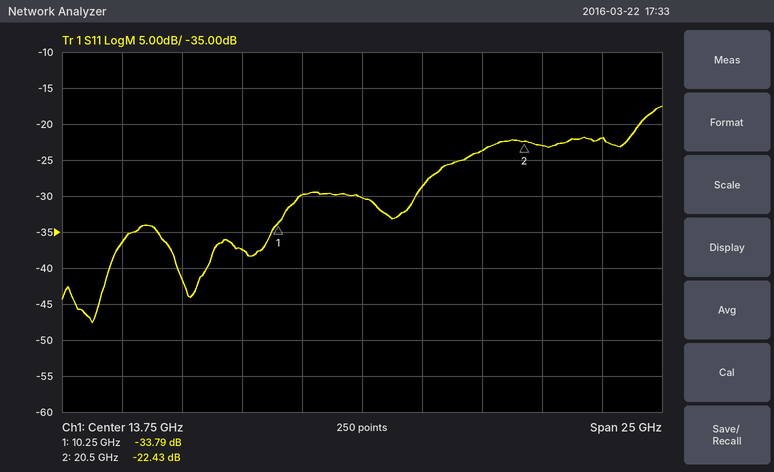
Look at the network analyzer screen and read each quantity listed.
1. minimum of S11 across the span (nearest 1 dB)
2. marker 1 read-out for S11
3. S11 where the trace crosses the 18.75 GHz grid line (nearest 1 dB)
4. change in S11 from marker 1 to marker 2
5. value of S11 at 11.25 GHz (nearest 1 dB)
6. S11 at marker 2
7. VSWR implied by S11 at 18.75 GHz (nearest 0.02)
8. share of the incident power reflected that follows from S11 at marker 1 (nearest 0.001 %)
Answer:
-48 dB
-33.79 dB
-24 dB
11.36 dB
-30 dB
-22.43 dB
1.14
0.042 %
